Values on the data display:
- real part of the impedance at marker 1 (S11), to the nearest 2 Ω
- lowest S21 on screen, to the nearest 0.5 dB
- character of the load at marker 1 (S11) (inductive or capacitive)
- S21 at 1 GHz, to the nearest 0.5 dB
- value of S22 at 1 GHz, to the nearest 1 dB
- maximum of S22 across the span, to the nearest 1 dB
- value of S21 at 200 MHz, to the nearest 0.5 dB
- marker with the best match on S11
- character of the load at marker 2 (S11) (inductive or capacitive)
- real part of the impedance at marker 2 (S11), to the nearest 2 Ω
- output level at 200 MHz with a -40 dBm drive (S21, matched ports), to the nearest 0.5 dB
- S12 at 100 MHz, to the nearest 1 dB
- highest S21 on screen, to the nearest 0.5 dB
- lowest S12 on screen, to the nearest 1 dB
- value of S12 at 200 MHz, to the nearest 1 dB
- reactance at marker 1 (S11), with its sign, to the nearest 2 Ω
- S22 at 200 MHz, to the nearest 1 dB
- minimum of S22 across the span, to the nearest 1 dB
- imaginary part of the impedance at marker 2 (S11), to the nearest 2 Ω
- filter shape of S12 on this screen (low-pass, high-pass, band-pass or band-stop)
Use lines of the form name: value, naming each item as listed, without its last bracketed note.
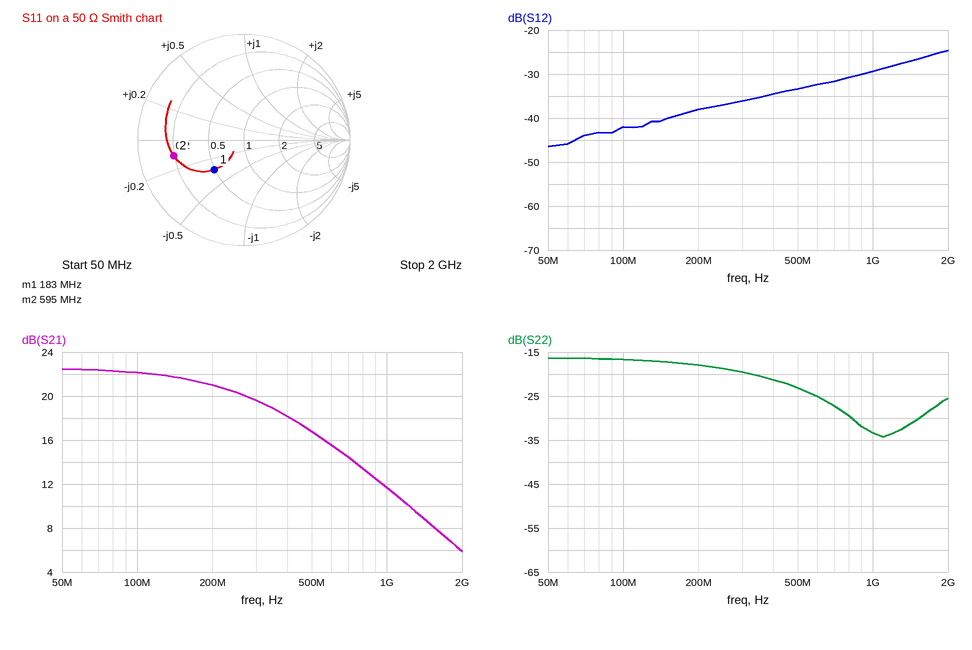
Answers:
real part of the impedance at marker 1 (S11), to the nearest 2 Ω: 24 Ω
lowest S21 on screen, to the nearest 0.5 dB: 6.0 dB
character of the load at marker 1 (S11): capacitive
S21 at 1 GHz, to the nearest 0.5 dB: 11.5 dB
value of S22 at 1 GHz, to the nearest 1 dB: -33 dB
maximum of S22 across the span, to the nearest 1 dB: -16 dB
value of S21 at 200 MHz, to the nearest 0.5 dB: 21.0 dB
marker with the best match on S11: marker 1
character of the load at marker 2 (S11): capacitive
real part of the impedance at marker 2 (S11), to the nearest 2 Ω: 10 Ω
output level at 200 MHz with a -40 dBm drive (S21, matched ports), to the nearest 0.5 dB: -19.0 dBm
S12 at 100 MHz, to the nearest 1 dB: -42 dB
highest S21 on screen, to the nearest 0.5 dB: 22.5 dB
lowest S12 on screen, to the nearest 1 dB: -46 dB
value of S12 at 200 MHz, to the nearest 1 dB: -38 dB
reactance at marker 1 (S11), with its sign, to the nearest 2 Ω: -16 Ω
S22 at 200 MHz, to the nearest 1 dB: -18 dB
minimum of S22 across the span, to the nearest 1 dB: -34 dB
imaginary part of the impedance at marker 2 (S11), to the nearest 2 Ω: -6 Ω
filter shape of S12 on this screen: high-pass
